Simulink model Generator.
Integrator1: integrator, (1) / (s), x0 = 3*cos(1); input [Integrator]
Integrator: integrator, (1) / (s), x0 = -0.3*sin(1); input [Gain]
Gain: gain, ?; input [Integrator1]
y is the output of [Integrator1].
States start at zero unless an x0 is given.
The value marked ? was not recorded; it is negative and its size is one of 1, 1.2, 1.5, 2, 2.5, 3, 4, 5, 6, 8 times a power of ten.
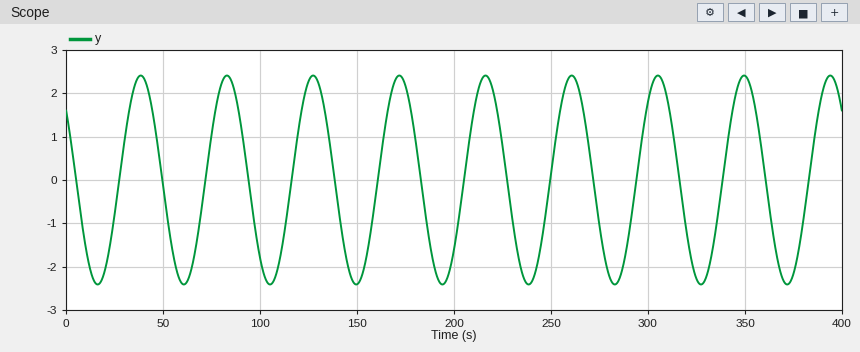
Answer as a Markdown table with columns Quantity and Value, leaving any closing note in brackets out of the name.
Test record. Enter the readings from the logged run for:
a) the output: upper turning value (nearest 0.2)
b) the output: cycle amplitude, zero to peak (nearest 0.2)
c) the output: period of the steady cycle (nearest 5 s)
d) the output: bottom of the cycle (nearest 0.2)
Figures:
| Quantity | Value |
|---|---|
| the output: upper turning value | 2.4 |
| the output: cycle amplitude, zero to peak | 2.4 |
| the output: period of the steady cycle | 45 s |
| the output: bottom of the cycle | -2.4 |
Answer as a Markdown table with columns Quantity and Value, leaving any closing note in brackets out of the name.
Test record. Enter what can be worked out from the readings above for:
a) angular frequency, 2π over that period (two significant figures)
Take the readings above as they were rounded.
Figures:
| Quantity | Value |
|---|---|
| angular frequency, 2π over that period | 0.14 rad/s |
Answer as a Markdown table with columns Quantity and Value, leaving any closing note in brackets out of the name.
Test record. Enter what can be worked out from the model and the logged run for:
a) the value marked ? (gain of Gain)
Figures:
| Quantity | Value |
|---|---|
| the value marked ? | -0.02 |
